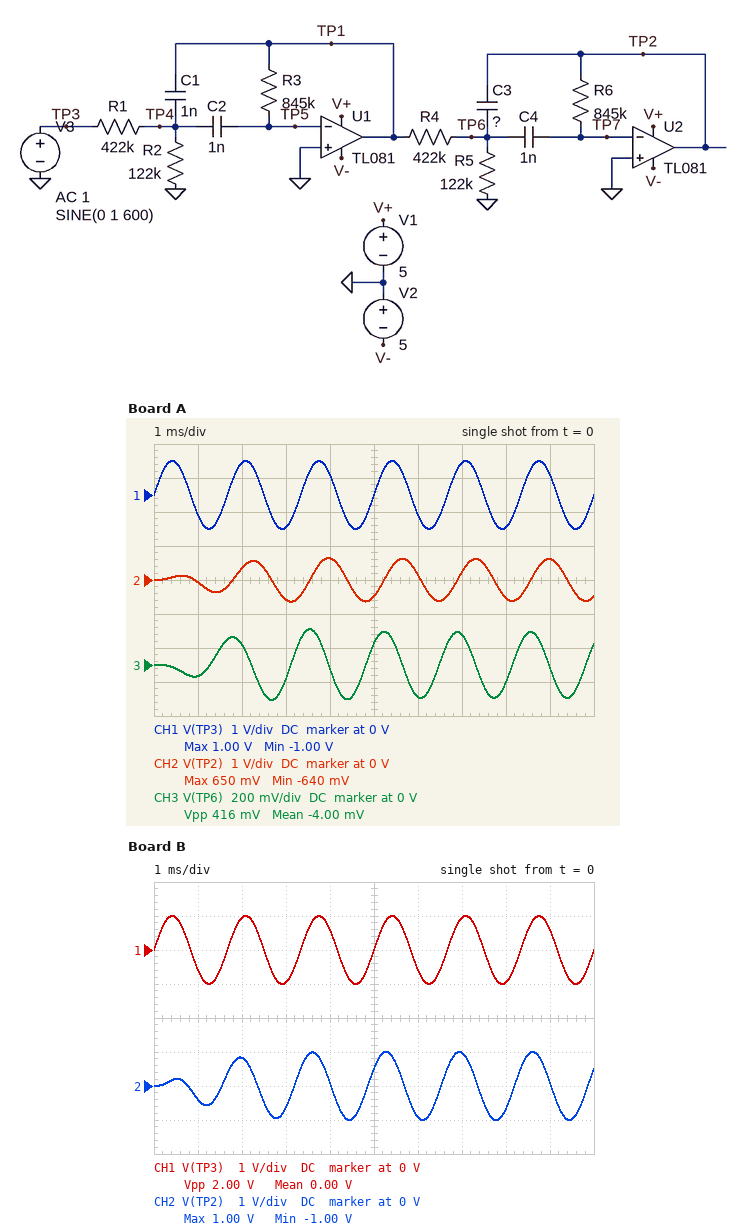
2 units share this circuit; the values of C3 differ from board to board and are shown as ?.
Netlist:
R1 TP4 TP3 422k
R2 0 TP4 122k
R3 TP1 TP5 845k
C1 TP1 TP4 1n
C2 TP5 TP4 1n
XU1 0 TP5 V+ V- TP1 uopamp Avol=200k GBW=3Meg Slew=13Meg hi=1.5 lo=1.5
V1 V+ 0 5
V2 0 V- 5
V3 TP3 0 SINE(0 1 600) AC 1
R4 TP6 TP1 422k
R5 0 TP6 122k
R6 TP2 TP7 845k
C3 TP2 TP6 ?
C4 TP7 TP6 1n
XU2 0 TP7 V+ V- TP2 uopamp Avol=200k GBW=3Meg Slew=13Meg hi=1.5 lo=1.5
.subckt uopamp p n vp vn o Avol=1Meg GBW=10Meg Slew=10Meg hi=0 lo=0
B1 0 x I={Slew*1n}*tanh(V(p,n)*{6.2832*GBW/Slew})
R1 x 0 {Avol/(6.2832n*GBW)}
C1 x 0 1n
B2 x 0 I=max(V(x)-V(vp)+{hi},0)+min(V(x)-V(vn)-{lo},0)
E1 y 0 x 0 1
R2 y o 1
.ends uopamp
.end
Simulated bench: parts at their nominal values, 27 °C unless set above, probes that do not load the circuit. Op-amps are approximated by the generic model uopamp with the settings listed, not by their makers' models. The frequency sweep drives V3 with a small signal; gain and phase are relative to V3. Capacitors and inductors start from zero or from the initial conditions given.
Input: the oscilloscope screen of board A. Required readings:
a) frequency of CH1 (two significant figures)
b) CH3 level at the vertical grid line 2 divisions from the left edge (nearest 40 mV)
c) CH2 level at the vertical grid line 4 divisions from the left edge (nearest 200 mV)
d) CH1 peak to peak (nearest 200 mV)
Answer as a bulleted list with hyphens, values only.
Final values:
- 600 Hz
- 120 mV
- 600 mV
- 2.0 V
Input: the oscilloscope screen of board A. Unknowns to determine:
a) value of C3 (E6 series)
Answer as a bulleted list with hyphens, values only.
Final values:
- 1.5 nF
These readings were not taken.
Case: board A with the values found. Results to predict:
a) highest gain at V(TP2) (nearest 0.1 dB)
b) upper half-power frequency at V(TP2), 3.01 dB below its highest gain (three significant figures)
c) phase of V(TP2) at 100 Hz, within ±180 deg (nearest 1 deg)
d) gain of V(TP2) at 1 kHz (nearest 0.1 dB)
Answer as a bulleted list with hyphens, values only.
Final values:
- -2.7 dB
- 646 Hz
- 164 deg
- -16.9 dB
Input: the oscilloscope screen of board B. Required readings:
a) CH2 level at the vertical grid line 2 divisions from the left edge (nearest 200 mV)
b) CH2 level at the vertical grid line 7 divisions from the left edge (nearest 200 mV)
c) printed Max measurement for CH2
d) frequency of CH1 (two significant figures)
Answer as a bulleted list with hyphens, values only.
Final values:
- 800 mV
- 1.0 V
- 1.00 V
- 600 Hz
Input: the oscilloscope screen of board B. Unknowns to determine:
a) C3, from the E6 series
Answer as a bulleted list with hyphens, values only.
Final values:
- 470 pF
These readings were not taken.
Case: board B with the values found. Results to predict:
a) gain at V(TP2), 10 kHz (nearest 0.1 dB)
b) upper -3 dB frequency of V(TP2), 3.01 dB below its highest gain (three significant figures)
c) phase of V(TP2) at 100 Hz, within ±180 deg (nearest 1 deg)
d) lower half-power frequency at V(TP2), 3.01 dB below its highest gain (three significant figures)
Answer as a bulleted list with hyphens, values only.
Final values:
- -50.3 dB
- 903 Hz
- 168 deg
- 502 Hz
